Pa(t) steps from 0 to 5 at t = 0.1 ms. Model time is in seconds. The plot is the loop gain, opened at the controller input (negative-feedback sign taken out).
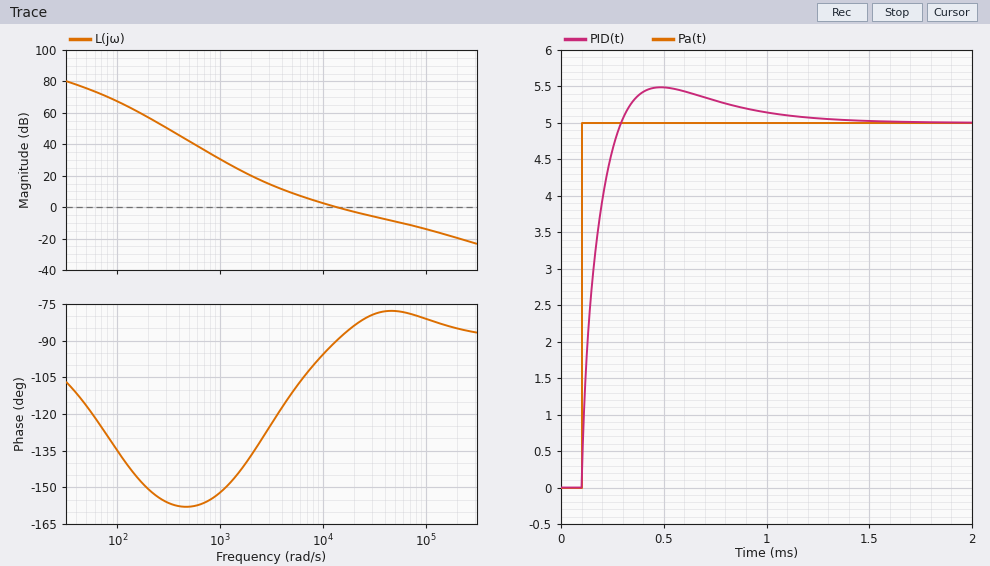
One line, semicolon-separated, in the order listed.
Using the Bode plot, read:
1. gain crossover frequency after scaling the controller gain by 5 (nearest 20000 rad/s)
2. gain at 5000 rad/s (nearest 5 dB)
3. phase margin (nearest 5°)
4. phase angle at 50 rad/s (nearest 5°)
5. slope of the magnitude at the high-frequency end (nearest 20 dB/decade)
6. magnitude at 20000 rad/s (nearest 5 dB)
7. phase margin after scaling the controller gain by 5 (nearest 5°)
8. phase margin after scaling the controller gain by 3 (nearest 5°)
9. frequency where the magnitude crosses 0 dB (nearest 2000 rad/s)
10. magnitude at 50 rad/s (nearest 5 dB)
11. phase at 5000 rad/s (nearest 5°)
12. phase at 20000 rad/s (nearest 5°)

100000 rad/s; 10 dB; 90°; -115°; -20 dB/decade; -5 dB; 100°; 100°; 14000 rad/s; 75 dB; -110°; -85°
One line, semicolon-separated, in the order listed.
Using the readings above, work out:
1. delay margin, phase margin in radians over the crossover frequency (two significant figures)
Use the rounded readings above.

0.00011 s
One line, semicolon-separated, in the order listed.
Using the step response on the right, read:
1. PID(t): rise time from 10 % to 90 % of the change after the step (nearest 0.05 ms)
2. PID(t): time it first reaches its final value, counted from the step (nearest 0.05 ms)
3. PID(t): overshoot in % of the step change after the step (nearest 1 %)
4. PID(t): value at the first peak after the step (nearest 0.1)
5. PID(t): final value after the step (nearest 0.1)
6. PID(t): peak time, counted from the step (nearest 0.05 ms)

0.15 ms; 0.20 ms; 10 %; 5.5; 5.0; 0.40 ms
